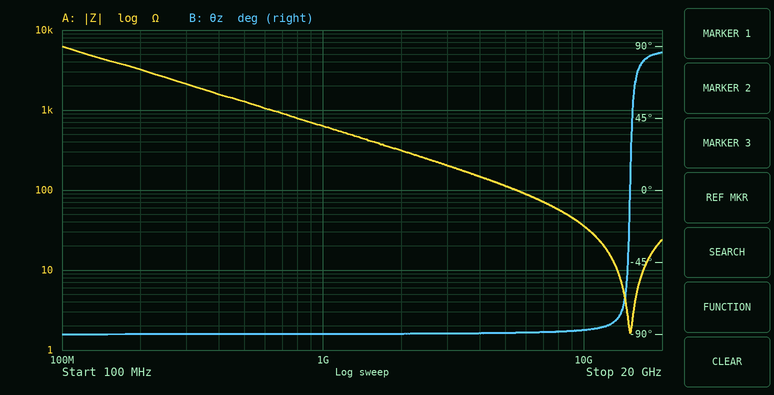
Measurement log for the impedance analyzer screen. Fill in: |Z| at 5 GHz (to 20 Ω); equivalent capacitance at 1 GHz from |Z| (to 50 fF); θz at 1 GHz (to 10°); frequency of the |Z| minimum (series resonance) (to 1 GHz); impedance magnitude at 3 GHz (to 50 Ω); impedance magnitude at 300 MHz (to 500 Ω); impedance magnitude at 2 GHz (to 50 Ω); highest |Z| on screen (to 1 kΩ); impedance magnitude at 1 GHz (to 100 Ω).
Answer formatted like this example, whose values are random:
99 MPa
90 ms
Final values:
120 Ω
250 fF
-90°
15 GHz
200 Ω
2.0 kΩ
300 Ω
6 kΩ
600 Ω
